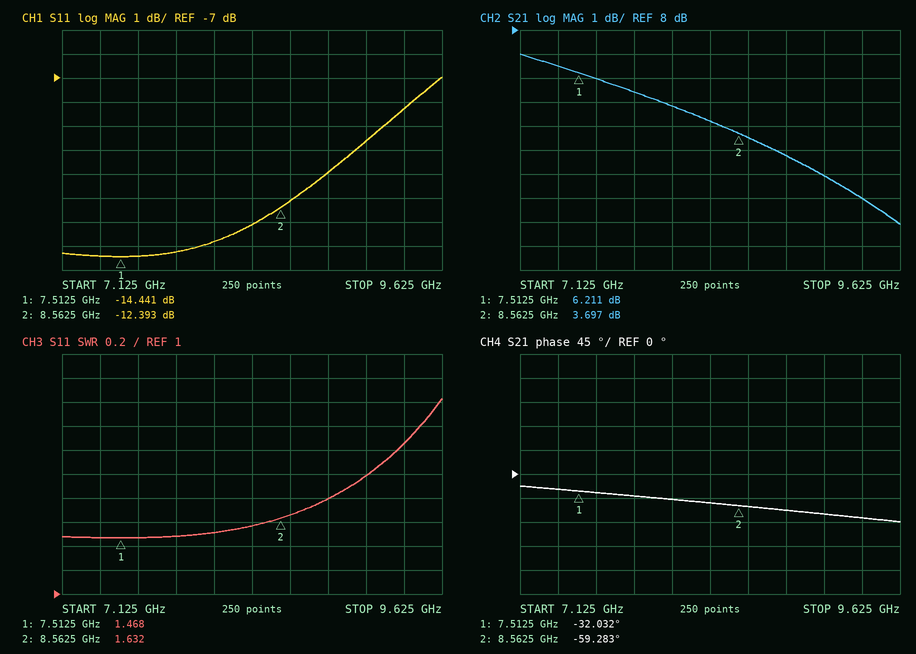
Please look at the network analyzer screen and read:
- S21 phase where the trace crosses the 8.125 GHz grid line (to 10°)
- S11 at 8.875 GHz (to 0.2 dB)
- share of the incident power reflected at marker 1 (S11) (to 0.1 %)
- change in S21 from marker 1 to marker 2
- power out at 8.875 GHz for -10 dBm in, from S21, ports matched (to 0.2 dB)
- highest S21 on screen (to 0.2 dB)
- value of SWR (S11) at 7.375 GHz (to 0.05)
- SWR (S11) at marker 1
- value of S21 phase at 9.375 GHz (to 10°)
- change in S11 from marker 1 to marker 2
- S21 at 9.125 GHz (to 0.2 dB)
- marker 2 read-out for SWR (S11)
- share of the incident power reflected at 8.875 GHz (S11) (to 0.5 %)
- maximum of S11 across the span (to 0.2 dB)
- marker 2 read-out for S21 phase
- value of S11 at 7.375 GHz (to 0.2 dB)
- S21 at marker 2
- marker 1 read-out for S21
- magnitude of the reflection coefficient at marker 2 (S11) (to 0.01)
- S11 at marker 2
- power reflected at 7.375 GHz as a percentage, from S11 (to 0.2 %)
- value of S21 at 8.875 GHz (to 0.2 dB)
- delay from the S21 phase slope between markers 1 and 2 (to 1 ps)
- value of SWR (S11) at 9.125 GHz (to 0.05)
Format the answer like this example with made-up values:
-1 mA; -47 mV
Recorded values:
-50°; -11.0 dB; 3.6 %; -2.514 dB; -7.2 dBm; 7.0 dB; 1.45; 1.468; -80°; 2.048 dB; 2.0 dB; 1.632; 8.0 %; -7.0 dB; -59.283°; -14.4 dB; 3.697 dB; 6.211 dB; 0.24; -12.393 dB; 3.6 %; 2.8 dB; 72 ps; 2.00
